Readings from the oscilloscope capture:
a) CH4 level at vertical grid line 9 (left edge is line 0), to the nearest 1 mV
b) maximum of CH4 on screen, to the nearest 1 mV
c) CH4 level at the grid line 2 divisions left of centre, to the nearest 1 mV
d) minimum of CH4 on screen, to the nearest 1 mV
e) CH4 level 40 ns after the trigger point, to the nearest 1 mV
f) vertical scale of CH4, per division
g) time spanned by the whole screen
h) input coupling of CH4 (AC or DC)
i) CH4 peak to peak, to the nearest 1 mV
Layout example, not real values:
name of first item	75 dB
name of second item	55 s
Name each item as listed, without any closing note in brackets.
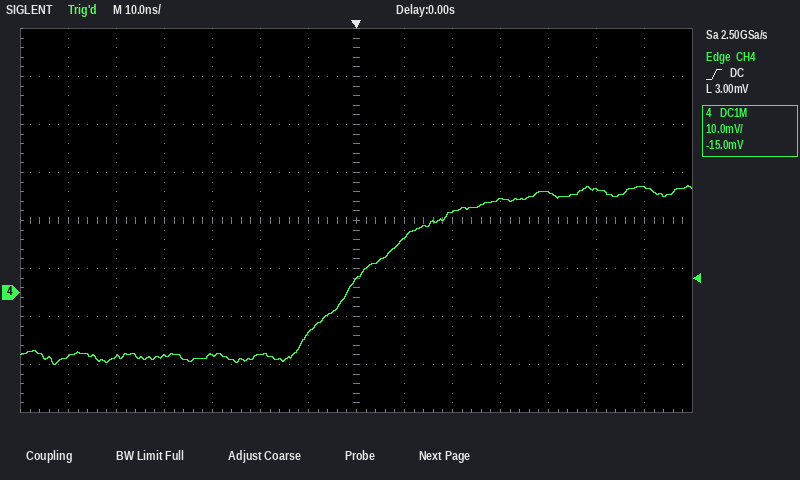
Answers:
CH4 level at vertical grid line 9 (left edge is line 0), to the nearest 1 mV	17 mV
maximum of CH4 on screen, to the nearest 1 mV	22 mV
CH4 level at the grid line 2 divisions left of centre, to the nearest 1 mV	-13 mV
minimum of CH4 on screen, to the nearest 1 mV	-15 mV
CH4 level 40 ns after the trigger point, to the nearest 1 mV	21 mV
vertical scale of CH4, per division	10 mV
time spanned by the whole screen	140 ns
input coupling of CH4	DC
CH4 peak to peak, to the nearest 1 mV	37 mV
